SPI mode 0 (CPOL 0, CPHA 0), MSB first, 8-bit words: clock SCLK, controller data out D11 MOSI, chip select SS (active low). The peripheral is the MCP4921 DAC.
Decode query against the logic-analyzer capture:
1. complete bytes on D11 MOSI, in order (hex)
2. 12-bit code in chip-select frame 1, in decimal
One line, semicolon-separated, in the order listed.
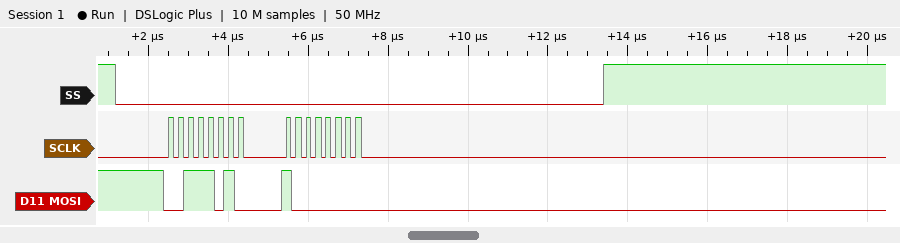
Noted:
0x3A 0x80; 2688
